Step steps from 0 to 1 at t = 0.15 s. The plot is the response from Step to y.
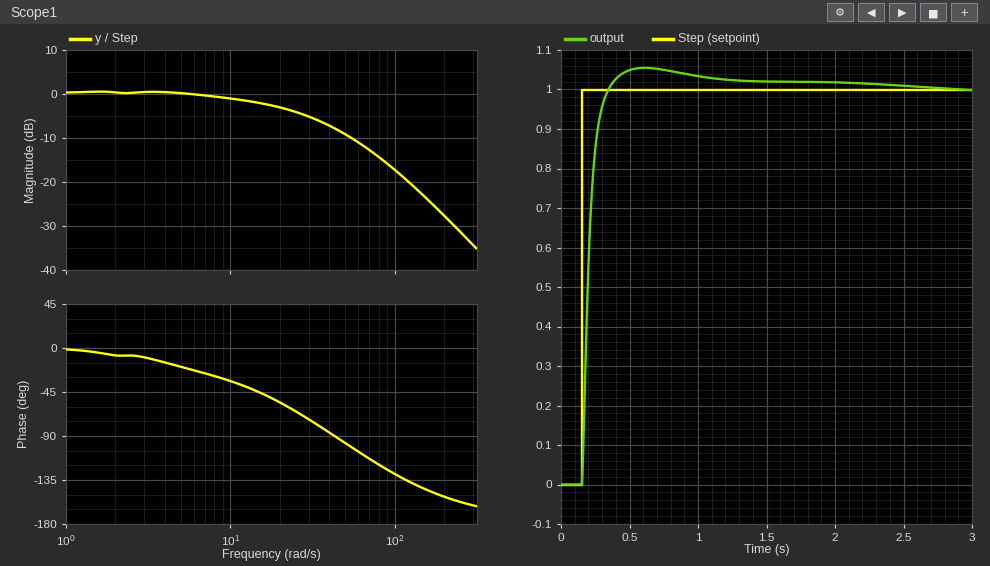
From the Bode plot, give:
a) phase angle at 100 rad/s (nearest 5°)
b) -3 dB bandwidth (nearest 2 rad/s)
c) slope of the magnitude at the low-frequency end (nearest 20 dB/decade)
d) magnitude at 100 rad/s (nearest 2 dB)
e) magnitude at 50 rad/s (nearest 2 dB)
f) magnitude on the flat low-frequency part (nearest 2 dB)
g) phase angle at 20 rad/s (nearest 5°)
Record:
-130°
18 rad/s
0 dB/decade
-18 dB
-10 dB
0 dB
-55°
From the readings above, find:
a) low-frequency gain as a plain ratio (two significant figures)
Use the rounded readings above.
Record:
1.0
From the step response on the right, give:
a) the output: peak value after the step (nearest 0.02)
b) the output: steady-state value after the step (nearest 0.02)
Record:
1.06
1.00
